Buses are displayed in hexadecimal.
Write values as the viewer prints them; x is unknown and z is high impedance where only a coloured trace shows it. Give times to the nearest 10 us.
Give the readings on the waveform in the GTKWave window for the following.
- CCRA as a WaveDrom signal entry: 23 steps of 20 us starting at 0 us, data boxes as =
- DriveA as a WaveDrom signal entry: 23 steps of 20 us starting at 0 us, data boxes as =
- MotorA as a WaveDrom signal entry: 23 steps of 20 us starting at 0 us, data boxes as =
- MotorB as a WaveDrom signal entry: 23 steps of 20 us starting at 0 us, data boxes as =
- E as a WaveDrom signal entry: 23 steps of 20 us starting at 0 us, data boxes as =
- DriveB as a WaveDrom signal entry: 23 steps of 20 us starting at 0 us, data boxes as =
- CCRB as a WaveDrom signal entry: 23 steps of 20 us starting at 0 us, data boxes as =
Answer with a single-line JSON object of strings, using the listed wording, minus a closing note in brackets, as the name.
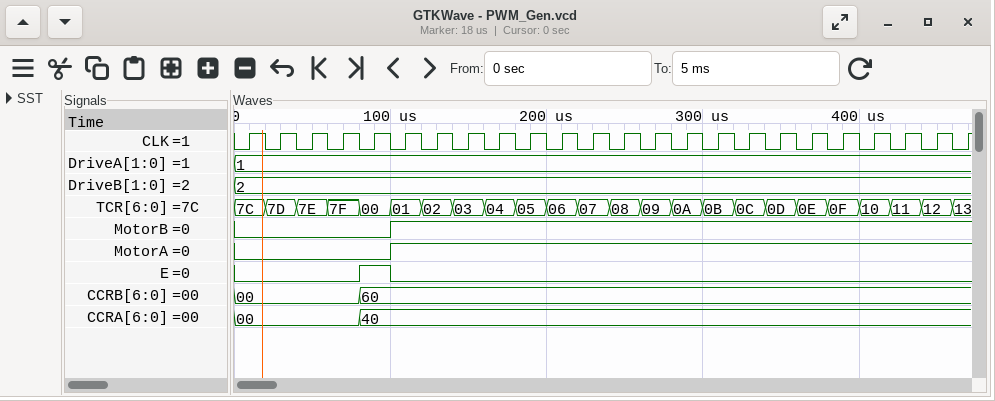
{"CCRA as a WaveDrom signal entry: 23 steps of 20 us starting at 0 us, data boxes as =": "{name: 'CCRA', wave: '=...=..................', data: '00 40'}", "DriveA as a WaveDrom signal entry: 23 steps of 20 us starting at 0 us, data boxes as =": "{name: 'DriveA', wave: '=......................', data: '1'}", "MotorA as a WaveDrom signal entry: 23 steps of 20 us starting at 0 us, data boxes as =": "{name: 'MotorA', wave: '0....1.................'}", "MotorB as a WaveDrom signal entry: 23 steps of 20 us starting at 0 us, data boxes as =": "{name: 'MotorB', wave: '0....1.................'}", "E as a WaveDrom signal entry: 23 steps of 20 us starting at 0 us, data boxes as =": "{name: 'E', wave: '0...10.................'}", "DriveB as a WaveDrom signal entry: 23 steps of 20 us starting at 0 us, data boxes as =": "{name: 'DriveB', wave: '=......................', data: '2'}", "CCRB as a WaveDrom signal entry: 23 steps of 20 us starting at 0 us, data boxes as =": "{name: 'CCRB', wave: '=...=..................', data: '00 60'}"}
